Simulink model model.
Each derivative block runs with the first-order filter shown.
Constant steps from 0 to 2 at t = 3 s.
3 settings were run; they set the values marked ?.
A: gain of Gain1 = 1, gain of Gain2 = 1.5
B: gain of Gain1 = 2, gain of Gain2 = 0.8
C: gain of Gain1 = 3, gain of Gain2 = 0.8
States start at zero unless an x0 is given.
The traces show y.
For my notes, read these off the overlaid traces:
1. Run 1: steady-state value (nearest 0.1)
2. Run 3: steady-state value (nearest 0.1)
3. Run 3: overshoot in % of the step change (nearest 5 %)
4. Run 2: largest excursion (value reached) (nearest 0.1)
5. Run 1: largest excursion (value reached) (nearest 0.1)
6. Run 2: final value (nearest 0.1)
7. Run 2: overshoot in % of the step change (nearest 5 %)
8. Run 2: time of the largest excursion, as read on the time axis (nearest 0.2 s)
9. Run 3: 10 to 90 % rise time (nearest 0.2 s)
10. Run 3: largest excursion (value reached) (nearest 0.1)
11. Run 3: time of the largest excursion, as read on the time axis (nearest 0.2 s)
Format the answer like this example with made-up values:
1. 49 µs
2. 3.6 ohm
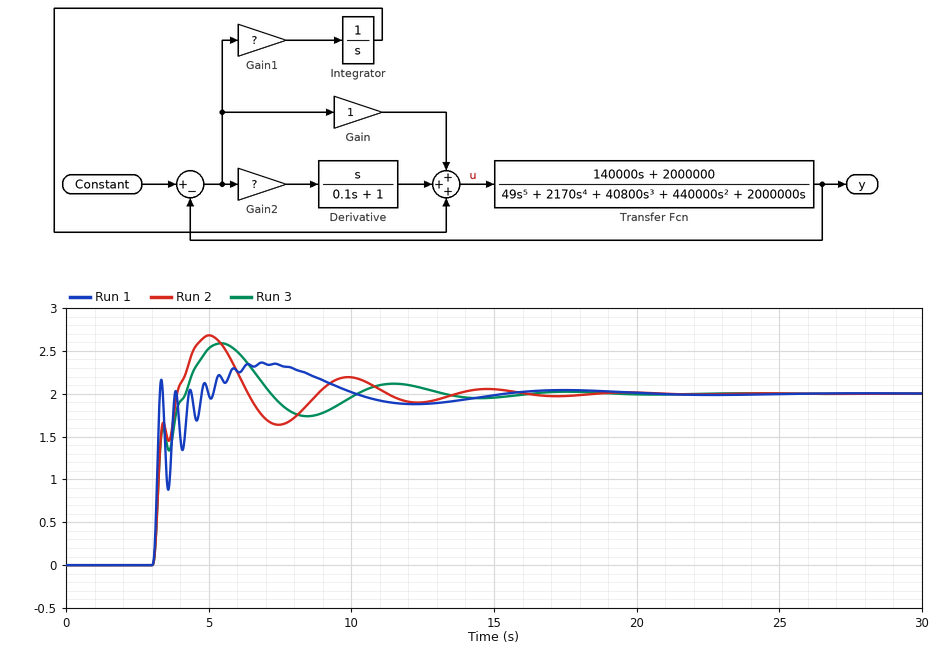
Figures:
1. 2.0
2. 2.0
3. 30 %
4. 2.7
5. 2.4
6. 2.0
7. 35 %
8. 5.0 s
9. 0.8 s
10. 2.6
11. 5.4 s
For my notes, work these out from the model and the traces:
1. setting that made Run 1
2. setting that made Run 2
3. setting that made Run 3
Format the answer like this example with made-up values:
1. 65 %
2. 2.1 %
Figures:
1. A
2. C
3. B
